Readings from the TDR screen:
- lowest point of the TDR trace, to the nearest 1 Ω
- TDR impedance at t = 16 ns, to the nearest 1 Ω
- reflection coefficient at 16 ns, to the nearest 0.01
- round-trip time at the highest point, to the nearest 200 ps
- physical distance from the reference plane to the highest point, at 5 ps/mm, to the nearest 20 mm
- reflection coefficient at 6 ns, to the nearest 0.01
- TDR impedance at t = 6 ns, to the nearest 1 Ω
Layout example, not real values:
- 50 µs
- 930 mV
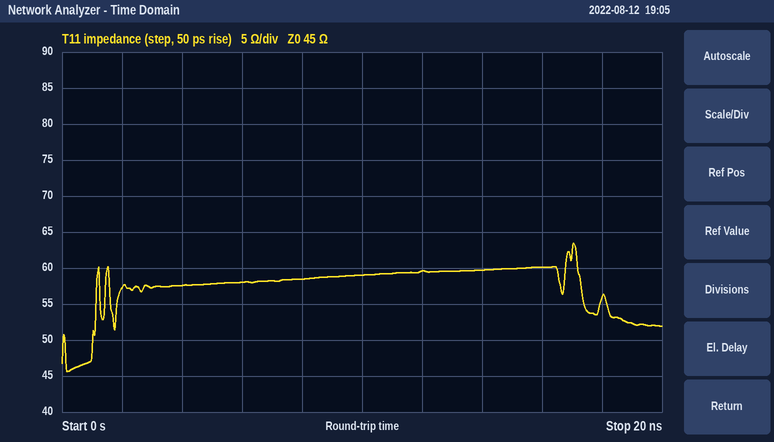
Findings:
- 46 Ω
- 60 Ω
- +0.14
- 17.0 ns
- 1.70 m
- +0.13
- 58 Ω
